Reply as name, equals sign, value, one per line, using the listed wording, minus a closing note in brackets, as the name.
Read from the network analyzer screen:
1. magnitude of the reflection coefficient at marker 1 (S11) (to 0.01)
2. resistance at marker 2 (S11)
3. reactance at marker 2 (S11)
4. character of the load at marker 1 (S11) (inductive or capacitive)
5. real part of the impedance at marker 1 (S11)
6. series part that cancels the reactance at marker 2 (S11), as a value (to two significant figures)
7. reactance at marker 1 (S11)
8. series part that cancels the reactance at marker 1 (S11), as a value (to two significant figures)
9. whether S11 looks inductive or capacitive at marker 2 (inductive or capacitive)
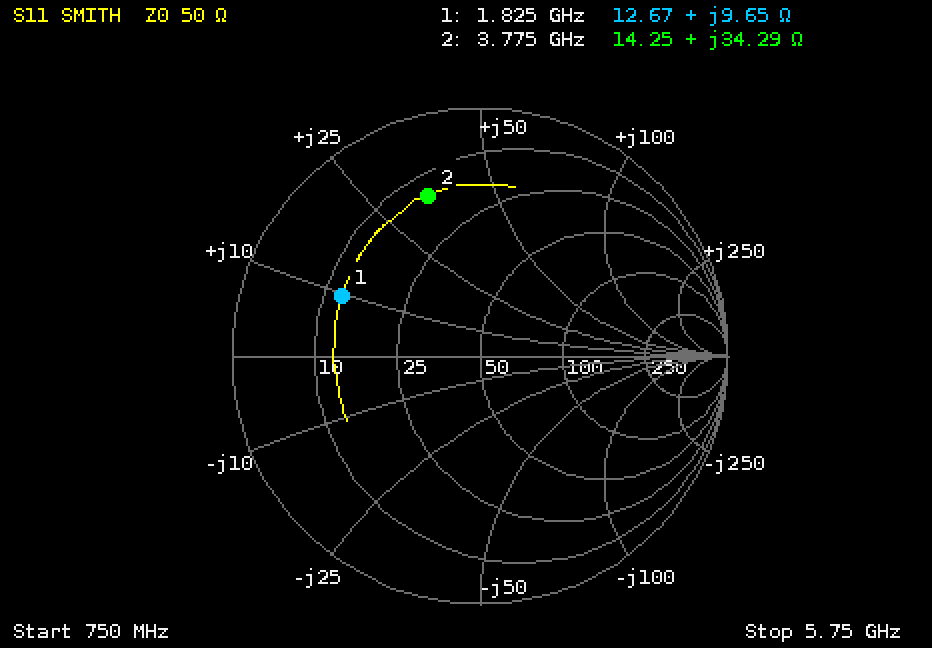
magnitude of the reflection coefficient at marker 1 (S11) = 0.61
resistance at marker 2 = 14.25 Ω
reactance at marker 2 = +34.29 Ω
character of the load at marker 1 (S11) = inductive
real part of the impedance at marker 1 = 12.67 Ω
series part that cancels the reactance at marker 2 (S11), as a value = 1.2 pF
reactance at marker 1 = +9.65 Ω
series part that cancels the reactance at marker 1 (S11), as a value = 9.0 pF
whether S11 looks inductive or capacitive at marker 2 = inductive
